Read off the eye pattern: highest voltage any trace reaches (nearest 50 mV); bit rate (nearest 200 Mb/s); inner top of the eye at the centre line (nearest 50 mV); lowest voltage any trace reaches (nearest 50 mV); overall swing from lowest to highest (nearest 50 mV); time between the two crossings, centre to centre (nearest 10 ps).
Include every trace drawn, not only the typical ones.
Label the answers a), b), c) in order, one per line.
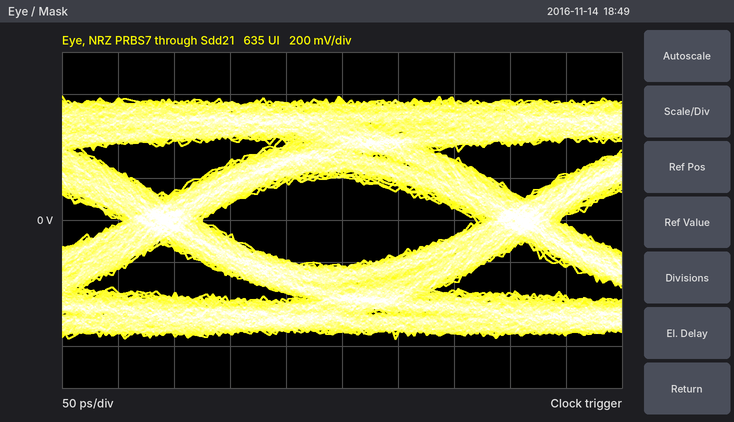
a) 600 mV
b) 3.2 Gb/s
c) 200 mV
d) -550 mV
e) 1.15 V
f) 320 ps
